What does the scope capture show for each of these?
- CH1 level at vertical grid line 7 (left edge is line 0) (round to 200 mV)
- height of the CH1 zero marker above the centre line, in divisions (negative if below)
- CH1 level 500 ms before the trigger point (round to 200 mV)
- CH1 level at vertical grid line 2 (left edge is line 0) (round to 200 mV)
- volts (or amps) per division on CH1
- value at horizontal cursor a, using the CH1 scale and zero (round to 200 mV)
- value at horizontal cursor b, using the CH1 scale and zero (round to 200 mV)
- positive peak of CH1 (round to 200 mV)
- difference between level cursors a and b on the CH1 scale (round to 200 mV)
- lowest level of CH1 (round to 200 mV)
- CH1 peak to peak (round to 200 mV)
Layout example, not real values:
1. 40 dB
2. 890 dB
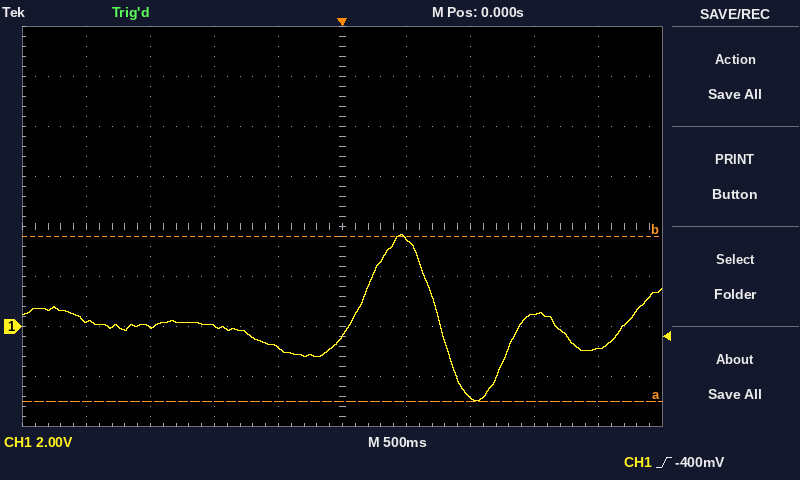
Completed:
1. -2.8 V
2. -2.0 div
3. -800 mV
4. 0.0 V
5. 2 V
6. -3.0 V
7. 3.6 V
8. 3.6 V
9. 6.6 V
10. -3.0 V
11. 6.6 V
